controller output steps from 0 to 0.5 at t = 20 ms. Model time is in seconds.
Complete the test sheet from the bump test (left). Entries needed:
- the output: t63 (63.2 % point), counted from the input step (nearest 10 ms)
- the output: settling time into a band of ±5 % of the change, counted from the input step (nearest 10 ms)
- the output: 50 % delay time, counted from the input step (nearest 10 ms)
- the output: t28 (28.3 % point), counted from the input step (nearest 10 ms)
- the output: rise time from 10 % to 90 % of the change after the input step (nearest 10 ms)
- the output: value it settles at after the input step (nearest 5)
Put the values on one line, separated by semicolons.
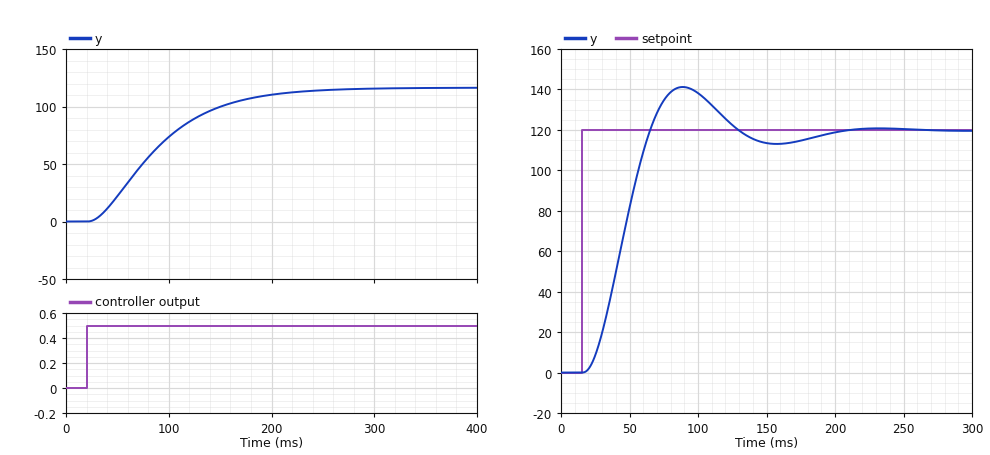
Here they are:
80 ms; 180 ms; 60 ms; 40 ms; 130 ms; 115
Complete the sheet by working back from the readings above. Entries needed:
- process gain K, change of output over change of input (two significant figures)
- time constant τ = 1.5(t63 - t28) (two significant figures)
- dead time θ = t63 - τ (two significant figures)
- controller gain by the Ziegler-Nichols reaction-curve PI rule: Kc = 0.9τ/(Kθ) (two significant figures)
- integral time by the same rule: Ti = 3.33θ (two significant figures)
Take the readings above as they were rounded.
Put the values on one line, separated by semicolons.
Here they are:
230; 60 ms; 20 ms; 0.012; 67 ms
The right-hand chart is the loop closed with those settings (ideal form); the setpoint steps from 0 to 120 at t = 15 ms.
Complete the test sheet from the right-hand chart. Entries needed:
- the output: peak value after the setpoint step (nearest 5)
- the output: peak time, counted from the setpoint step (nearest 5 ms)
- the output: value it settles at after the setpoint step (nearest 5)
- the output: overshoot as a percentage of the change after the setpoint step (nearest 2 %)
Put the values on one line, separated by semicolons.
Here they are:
140; 75 ms; 120; 18 %
